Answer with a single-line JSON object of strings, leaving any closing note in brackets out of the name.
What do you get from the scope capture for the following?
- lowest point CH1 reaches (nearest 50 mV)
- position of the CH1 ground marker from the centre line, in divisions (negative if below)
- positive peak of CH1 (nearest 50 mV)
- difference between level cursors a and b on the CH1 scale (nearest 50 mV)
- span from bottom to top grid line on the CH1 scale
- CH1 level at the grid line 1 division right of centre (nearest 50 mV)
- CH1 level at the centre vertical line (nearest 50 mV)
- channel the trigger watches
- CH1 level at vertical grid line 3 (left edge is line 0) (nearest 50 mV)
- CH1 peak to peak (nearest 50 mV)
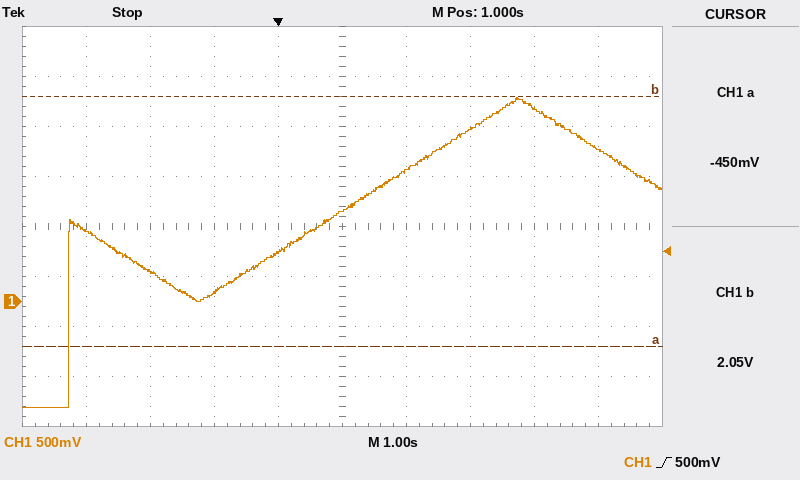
{"lowest point CH1 reaches": "-1.05 V", "position of the CH1 ground marker from the centre line, in divisions": "-1.5 div", "positive peak of CH1": "2.05 V", "difference between level cursors a and b on the CH1 scale": "2.50 V", "span from bottom to top grid line on the CH1 scale": "4 V", "CH1 level at the grid line 1 division right of centre": "1.30 V", "CH1 level at the centre vertical line": "900 mV", "channel the trigger watches": "CH1", "CH1 level at vertical grid line 3 (left edge is line 0)": "100 mV", "CH1 peak to peak": "3.10 V"}
